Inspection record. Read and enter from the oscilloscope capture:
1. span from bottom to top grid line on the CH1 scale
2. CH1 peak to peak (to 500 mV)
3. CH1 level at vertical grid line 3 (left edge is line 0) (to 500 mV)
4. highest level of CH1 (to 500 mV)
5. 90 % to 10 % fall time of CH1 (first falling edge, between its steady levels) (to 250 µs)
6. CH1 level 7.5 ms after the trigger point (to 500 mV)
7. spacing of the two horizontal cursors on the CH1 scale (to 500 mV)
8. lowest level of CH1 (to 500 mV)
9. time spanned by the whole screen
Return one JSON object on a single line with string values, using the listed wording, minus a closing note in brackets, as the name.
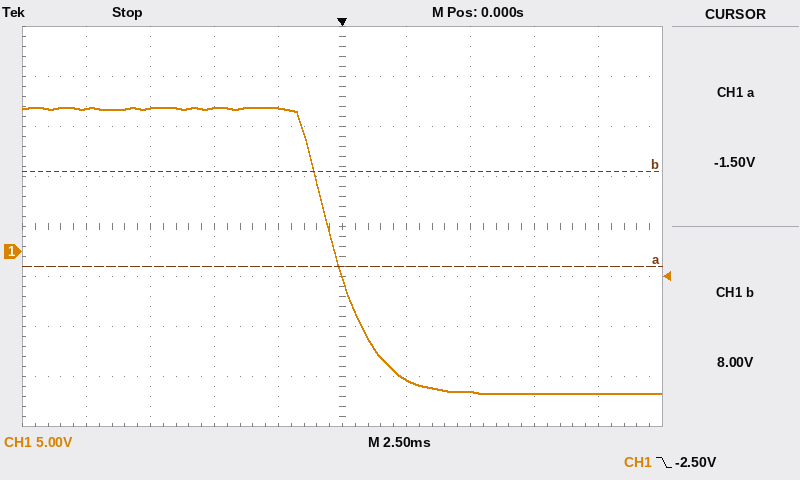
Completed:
{"span from bottom to top grid line on the CH1 scale": "40 V", "CH1 peak to peak": "28.5 V", "CH1 level at vertical grid line 3 (left edge is line 0)": "14.5 V", "highest level of CH1": "14.5 V", "90 % to 10 % fall time of CH1 (first falling edge, between its steady levels)": "3.25 ms", "CH1 level 7.5 ms after the trigger point": "-14.0 V", "spacing of the two horizontal cursors on the CH1 scale": "9.5 V", "lowest level of CH1": "-14.0 V", "time spanned by the whole screen": "25 ms"}
